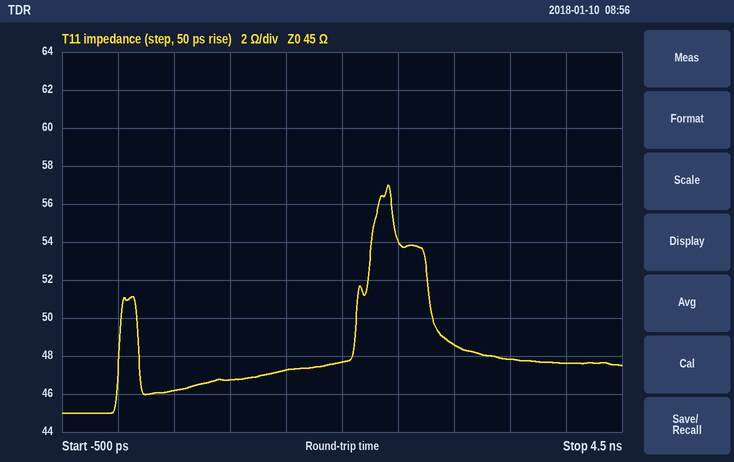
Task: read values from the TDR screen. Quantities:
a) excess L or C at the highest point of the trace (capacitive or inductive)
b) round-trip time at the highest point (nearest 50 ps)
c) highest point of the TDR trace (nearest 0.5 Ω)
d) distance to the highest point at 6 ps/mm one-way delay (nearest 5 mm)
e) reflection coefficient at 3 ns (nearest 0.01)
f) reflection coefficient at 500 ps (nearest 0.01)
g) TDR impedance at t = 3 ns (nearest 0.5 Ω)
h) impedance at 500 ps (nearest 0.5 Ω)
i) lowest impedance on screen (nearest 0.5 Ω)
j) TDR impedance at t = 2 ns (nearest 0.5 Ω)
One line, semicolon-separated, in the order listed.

inductive; 2.40 ns; 57.0 Ω; 200 mm; +0.04; +0.01; 48.5 Ω; 46.0 Ω; 45.0 Ω; 47.5 Ω
